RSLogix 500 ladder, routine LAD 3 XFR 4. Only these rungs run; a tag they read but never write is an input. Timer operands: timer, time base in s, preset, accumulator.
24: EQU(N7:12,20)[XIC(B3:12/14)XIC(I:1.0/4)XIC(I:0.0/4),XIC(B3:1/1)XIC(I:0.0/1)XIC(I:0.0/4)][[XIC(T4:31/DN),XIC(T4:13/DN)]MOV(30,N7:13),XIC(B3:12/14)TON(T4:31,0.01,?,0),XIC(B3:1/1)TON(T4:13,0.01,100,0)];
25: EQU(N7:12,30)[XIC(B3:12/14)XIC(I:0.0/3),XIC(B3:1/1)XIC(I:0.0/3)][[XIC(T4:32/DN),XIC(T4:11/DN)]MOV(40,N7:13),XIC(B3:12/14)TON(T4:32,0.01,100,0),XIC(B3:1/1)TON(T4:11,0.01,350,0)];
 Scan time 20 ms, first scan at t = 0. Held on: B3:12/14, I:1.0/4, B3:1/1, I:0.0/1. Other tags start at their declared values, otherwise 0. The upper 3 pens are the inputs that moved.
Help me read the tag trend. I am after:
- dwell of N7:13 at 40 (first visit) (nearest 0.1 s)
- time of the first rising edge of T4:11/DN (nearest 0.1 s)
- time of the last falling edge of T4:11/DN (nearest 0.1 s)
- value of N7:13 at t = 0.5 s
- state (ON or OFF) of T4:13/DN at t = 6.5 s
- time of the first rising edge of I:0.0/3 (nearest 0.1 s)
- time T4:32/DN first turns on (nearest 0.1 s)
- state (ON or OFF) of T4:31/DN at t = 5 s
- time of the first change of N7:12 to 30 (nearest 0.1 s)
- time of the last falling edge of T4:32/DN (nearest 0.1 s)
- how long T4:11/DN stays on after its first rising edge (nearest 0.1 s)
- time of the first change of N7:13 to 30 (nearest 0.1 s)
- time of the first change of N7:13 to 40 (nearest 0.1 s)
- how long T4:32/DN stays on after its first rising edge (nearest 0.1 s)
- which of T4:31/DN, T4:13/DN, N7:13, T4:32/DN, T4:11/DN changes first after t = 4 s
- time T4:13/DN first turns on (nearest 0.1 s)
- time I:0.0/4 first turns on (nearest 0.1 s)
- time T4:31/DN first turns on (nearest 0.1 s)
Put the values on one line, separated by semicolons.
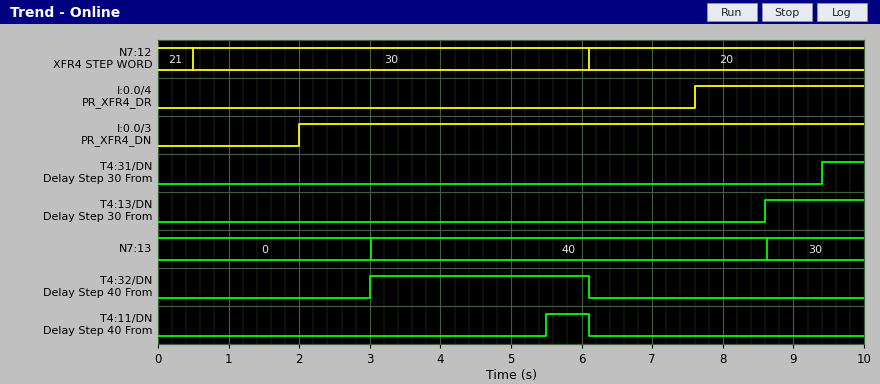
5.6 s; 5.5 s; 6.1 s; 0; OFF; 2.0 s; 3.0 s; OFF; 0.5 s; 6.1 s; 0.6 s; 8.6 s; 3.0 s; 3.1 s; T4:11/DN; 8.6 s; 7.6 s; 9.4 s
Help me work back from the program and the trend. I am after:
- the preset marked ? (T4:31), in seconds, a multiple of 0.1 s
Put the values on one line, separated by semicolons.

1.8 s
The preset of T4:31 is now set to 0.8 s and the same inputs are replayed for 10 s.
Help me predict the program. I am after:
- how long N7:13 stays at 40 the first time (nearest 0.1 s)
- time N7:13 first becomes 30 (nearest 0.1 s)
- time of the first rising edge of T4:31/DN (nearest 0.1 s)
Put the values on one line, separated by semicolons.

5.4 s; 8.4 s; 8.4 s
